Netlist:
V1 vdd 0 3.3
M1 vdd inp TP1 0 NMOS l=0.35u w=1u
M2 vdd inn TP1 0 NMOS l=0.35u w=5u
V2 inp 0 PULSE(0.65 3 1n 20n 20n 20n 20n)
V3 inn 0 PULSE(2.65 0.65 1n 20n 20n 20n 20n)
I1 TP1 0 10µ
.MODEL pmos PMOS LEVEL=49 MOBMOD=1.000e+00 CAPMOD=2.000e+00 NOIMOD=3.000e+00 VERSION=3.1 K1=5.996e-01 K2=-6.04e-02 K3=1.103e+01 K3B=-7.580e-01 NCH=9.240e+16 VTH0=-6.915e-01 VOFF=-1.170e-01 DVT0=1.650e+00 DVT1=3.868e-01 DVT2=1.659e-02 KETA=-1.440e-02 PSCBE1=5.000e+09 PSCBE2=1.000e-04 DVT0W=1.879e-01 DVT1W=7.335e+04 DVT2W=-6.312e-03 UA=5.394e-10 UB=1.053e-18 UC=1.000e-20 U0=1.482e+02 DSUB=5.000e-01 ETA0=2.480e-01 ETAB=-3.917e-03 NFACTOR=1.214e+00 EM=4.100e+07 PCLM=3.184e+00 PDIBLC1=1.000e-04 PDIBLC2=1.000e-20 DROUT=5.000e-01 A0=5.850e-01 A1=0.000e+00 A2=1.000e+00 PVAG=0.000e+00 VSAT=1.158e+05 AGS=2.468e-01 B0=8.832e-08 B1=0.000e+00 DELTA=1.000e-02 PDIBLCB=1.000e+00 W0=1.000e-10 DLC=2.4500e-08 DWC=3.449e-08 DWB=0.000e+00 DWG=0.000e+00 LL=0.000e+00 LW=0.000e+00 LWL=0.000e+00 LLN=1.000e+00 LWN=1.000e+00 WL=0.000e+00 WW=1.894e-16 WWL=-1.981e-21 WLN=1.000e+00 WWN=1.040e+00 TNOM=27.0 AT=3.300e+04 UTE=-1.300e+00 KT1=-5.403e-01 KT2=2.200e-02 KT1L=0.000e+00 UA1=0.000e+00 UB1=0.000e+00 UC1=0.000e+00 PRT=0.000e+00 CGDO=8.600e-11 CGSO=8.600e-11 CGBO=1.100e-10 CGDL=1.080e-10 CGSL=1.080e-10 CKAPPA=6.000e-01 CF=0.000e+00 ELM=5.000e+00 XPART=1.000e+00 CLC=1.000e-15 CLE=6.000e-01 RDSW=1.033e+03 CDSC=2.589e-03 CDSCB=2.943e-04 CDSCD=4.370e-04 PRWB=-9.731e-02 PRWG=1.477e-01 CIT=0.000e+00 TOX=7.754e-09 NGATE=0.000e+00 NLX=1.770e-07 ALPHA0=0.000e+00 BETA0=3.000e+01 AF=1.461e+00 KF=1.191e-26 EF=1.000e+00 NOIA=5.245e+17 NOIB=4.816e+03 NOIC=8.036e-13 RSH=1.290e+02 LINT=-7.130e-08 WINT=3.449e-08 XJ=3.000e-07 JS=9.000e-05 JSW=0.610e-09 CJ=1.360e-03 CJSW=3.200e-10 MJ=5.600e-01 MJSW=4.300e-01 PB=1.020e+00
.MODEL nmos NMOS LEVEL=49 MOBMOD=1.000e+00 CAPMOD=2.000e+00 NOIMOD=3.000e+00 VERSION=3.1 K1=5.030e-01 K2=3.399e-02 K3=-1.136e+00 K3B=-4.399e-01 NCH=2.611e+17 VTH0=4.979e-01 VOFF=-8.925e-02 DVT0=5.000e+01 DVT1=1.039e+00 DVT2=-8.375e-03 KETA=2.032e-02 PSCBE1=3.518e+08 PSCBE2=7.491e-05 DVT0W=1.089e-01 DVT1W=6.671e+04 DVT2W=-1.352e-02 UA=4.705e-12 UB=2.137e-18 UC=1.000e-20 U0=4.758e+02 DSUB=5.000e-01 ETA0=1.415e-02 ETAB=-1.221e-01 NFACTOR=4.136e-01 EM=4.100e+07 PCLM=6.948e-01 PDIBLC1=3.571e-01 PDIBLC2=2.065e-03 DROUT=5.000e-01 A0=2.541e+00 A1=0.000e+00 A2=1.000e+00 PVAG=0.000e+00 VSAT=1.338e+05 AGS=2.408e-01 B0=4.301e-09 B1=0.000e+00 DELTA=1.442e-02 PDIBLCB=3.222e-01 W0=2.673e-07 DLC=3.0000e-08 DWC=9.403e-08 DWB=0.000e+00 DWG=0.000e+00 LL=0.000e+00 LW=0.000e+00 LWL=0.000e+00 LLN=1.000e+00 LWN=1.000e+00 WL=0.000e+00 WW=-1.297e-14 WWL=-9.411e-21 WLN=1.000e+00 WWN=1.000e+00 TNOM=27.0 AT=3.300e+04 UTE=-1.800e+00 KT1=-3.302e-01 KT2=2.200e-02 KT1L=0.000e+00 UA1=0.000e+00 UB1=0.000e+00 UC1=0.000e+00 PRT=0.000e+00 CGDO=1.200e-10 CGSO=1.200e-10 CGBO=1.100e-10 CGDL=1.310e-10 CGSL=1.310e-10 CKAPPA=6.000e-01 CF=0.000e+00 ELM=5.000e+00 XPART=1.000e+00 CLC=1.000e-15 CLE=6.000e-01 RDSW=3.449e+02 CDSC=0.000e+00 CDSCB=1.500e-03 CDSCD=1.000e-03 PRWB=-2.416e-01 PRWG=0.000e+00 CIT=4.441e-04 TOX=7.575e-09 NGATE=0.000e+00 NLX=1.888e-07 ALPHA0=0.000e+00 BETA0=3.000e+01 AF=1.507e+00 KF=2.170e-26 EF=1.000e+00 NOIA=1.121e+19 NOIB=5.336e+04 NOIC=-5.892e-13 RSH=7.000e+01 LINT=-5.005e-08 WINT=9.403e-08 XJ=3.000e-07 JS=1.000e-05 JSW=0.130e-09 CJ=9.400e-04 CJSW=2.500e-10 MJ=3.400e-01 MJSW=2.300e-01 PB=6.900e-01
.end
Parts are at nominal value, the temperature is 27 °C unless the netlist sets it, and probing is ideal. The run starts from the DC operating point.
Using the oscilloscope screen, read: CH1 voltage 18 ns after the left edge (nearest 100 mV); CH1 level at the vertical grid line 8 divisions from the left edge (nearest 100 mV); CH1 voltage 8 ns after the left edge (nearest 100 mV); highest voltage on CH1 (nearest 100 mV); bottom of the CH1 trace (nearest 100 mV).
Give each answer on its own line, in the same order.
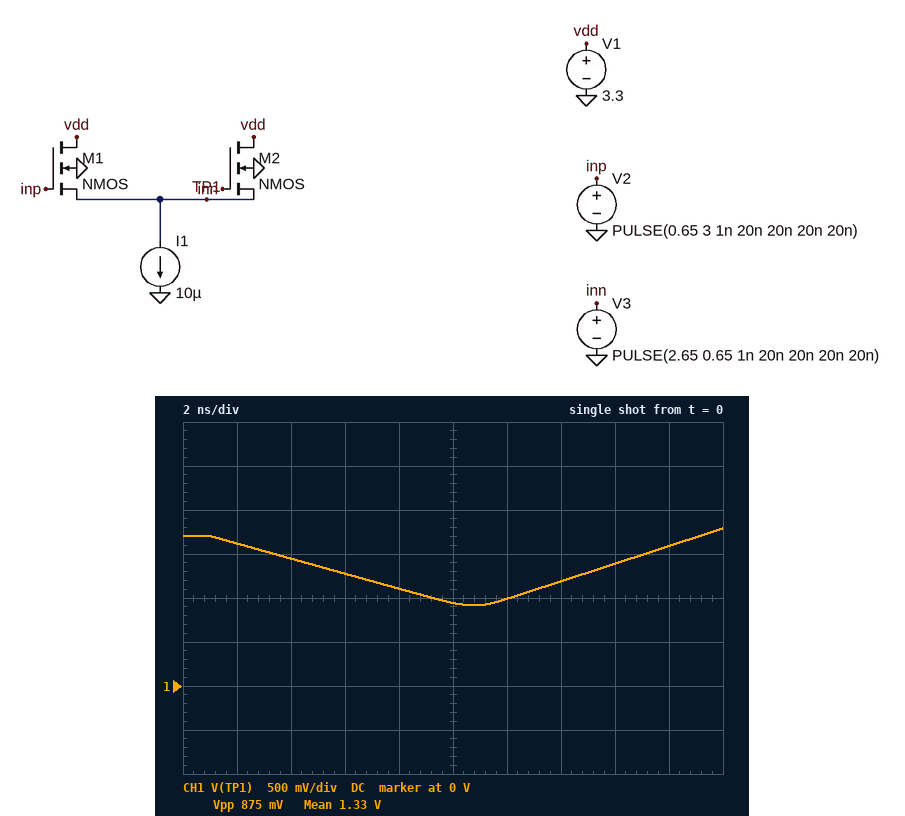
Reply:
1.6 V
1.4 V
1.1 V
1.8 V
900 mV
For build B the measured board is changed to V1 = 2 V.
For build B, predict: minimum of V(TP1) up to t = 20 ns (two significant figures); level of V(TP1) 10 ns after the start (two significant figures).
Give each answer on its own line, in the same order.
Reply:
900 mV
930 mV
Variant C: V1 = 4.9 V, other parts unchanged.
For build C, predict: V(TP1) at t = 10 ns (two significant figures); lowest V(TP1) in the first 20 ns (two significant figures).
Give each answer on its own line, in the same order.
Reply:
980 mV
950 mV
